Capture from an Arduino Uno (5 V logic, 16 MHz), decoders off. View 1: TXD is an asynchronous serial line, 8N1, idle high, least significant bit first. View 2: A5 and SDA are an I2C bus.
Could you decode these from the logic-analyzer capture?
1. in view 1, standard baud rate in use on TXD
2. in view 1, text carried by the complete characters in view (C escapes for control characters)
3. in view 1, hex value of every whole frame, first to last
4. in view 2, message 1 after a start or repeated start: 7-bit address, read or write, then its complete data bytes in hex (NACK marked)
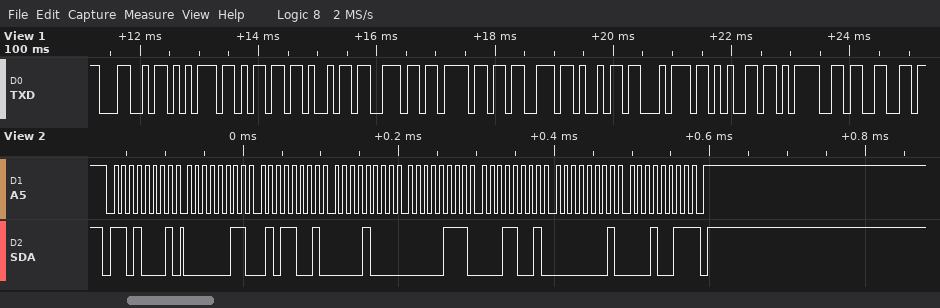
9600 baud
"Luminosite=3"
4C 75 6D 69 6E 6F 73 69 74 65 3D 33
0x68 read: 03 59 08 07 19 01 13 NACK
